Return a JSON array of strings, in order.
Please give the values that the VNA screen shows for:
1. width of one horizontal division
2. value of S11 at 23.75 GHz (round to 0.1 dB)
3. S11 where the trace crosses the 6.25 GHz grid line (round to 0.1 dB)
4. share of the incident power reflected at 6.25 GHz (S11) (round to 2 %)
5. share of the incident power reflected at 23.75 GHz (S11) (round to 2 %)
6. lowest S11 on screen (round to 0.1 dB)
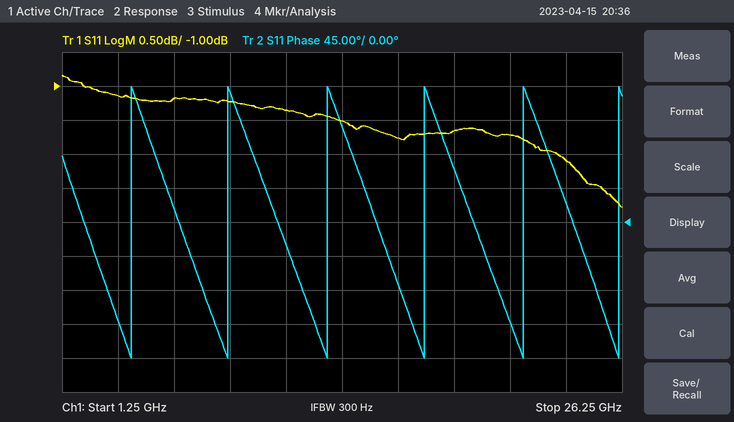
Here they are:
["2.5 GHz", "-2.1 dB", "-1.2 dB", "76 %", "62 %", "-2.8 dB"]
